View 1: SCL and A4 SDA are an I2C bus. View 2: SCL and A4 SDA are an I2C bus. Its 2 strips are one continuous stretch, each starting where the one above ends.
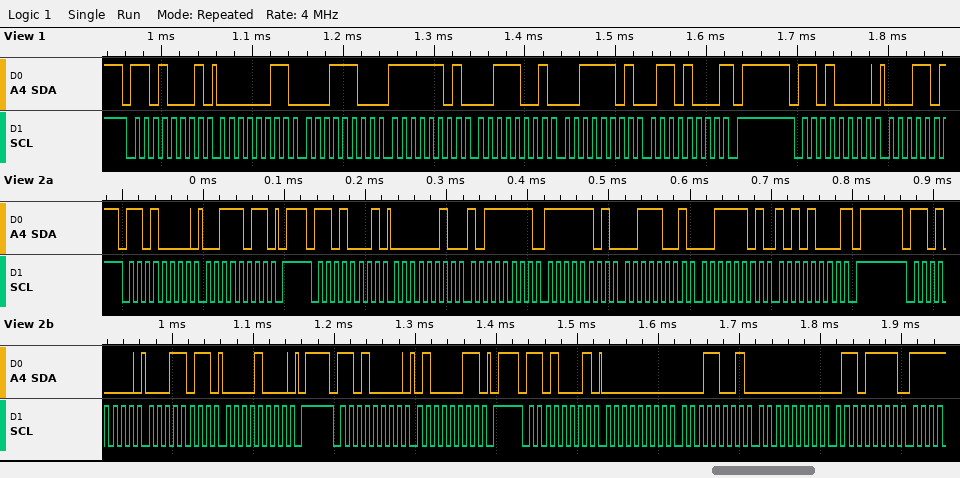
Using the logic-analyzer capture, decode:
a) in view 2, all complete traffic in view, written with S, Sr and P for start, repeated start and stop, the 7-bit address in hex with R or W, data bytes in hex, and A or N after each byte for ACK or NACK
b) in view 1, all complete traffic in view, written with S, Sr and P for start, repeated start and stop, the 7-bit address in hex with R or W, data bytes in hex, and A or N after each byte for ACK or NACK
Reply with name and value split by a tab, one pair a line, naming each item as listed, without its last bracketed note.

in view 2, all complete traffic in view, written with S, Sr and P for start, repeated start and stop, the 7-bit address in hex with R or W, data bytes in hex, and A or N after each byte for ACK or NACK	S 68W A 3B A P S 68R A 02 A BF A FD A 39 A 3D A A8 N P S 68W A 1B A 08 A P S 68W A 43 A P S 68R A 00 A 19 A 00 A 6F A
in view 1, all complete traffic in view, written with S, Sr and P for start, repeated start and stop, the 7-bit address in hex with R or W, data bytes in hex, and A or N after each byte for ACK or NACK	S 68R A 03 A 1C A FD A 39 A 3D A 68 N P S 68W A
